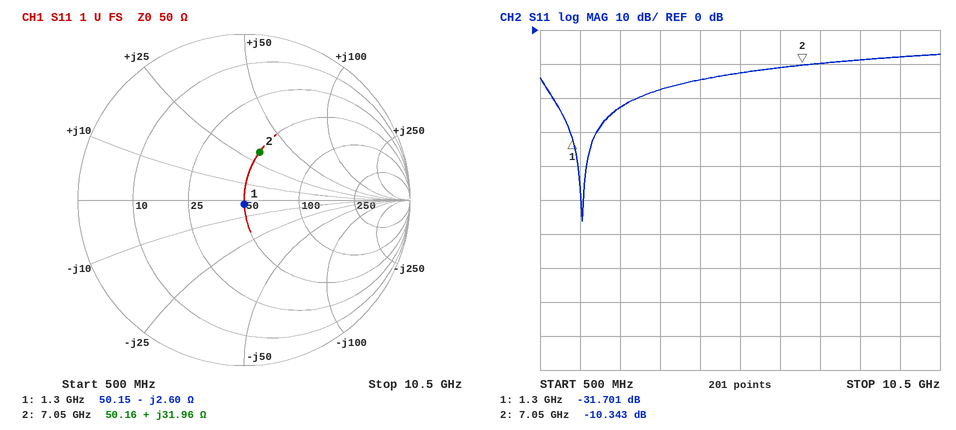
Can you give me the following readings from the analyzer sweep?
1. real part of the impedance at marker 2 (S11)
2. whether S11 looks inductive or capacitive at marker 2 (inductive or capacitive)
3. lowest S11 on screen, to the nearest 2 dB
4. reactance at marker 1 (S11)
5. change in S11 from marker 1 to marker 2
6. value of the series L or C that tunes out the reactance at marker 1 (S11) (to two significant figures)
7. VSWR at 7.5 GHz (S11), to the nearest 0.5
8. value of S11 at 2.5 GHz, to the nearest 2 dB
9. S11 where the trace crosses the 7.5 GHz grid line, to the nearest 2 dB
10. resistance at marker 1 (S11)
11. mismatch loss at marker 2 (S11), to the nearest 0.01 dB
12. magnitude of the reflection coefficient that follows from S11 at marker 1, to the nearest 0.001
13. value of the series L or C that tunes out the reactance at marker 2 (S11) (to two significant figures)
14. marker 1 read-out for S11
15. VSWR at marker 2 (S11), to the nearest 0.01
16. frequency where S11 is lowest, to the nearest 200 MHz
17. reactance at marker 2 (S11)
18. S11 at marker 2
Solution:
50.16 Ω
inductive
-56 dB
-2.60 Ω
21.358 dB
320 pH
2.0
-22 dB
-10 dB
50.15 Ω
0.42 dB
0.026
710 fF
-31.701 dB
1.87
1.6 GHz
+31.96 Ω
-10.343 dB
